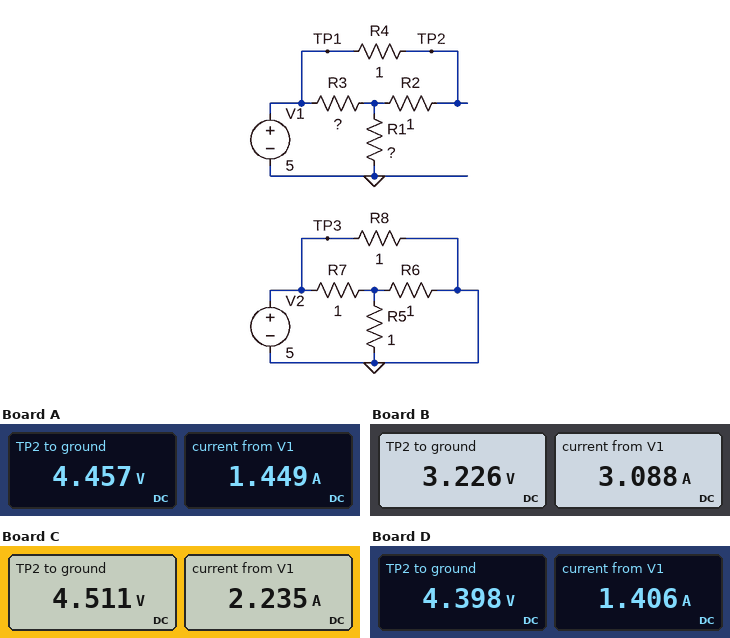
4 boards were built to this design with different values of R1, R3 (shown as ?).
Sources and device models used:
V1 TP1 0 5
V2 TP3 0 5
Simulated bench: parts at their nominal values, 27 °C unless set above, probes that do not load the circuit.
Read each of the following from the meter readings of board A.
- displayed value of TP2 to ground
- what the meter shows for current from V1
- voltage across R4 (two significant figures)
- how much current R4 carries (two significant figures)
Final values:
4.457 V
1.449 A
540 mV
540 mA
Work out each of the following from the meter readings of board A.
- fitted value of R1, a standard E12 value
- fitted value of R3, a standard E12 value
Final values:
2.7 Ω
1.2 Ω
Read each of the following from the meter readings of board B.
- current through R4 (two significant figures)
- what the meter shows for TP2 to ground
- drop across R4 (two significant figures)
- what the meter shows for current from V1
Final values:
1.8 A
3.226 V
1.8 V
3.088 A
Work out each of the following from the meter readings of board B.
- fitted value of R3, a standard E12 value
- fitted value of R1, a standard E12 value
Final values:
2.7 Ω
0.47 Ω
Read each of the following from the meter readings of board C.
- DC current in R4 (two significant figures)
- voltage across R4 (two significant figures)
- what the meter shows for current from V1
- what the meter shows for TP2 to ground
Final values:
490 mA
490 mV
2.235 A
4.511 V
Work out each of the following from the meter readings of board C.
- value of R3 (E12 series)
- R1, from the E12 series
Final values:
0.56 Ω
1.8 Ω
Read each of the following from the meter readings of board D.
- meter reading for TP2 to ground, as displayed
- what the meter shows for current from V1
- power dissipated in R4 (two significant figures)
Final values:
4.398 V
1.406 A
360 mW
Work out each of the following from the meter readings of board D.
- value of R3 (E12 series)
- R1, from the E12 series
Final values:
1.5 Ω
2.7 Ω
